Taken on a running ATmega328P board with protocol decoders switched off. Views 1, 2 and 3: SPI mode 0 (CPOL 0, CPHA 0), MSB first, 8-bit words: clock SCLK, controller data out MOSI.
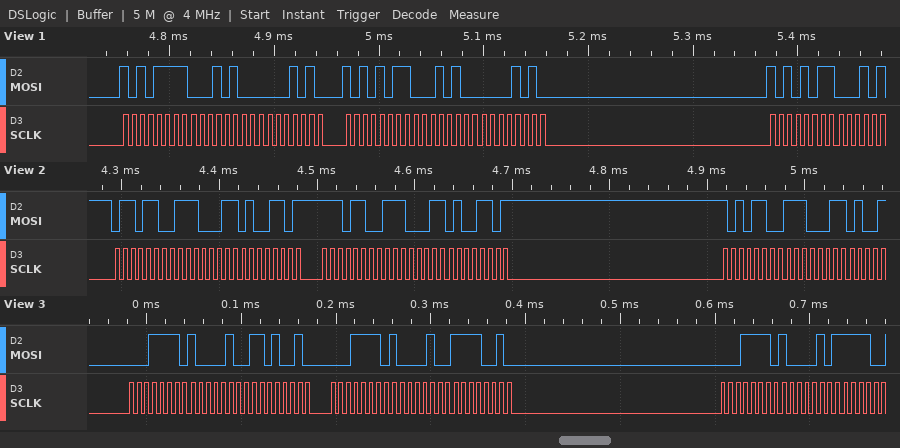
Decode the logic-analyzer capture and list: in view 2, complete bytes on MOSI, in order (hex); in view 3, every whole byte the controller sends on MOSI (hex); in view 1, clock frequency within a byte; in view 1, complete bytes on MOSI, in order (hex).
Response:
6C E3 4D EC E3 4D AC E3
1E 84 D2 1E 84 F2 1E 85
125 kHz
AF 14 0A AB 14 0A AB
